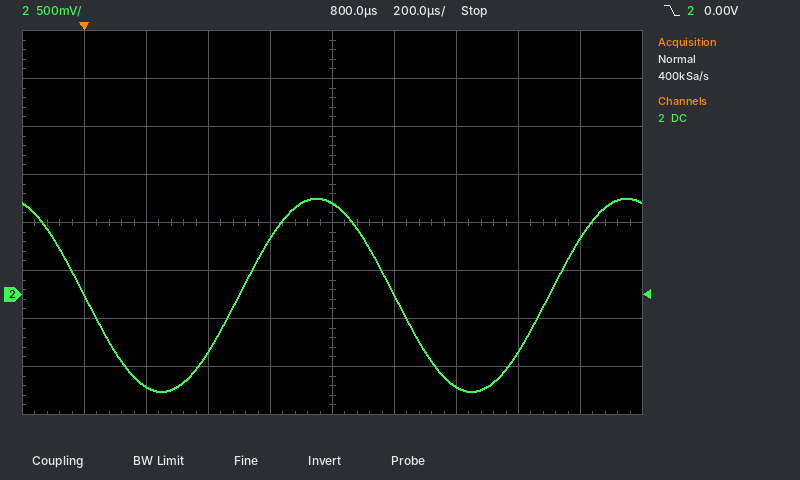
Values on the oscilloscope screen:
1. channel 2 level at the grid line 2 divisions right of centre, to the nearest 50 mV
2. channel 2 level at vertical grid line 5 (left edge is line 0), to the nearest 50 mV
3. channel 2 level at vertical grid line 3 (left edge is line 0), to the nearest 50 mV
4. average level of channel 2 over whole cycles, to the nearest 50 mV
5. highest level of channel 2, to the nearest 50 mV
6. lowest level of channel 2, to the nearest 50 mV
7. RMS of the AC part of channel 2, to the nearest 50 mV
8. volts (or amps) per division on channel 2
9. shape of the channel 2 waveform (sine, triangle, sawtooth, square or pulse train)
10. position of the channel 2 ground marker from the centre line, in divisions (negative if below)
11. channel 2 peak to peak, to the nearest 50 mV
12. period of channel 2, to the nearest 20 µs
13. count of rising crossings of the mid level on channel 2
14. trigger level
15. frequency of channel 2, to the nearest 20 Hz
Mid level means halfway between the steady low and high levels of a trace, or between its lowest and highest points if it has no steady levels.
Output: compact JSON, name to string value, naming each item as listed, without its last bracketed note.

{"channel 2 level at the grid line 2 divisions right of centre, to the nearest 50 mV": "-950 mV", "channel 2 level at vertical grid line 5 (left edge is line 0), to the nearest 50 mV": "950 mV", "channel 2 level at vertical grid line 3 (left edge is line 0), to the nearest 50 mV": "-600 mV", "average level of channel 2 over whole cycles, to the nearest 50 mV": "0 mV", "highest level of channel 2, to the nearest 50 mV": "1.00 V", "lowest level of channel 2, to the nearest 50 mV": "-1.00 V", "RMS of the AC part of channel 2, to the nearest 50 mV": "700 mV", "volts (or amps) per division on channel 2": "500 mV", "shape of the channel 2 waveform": "sine", "position of the channel 2 ground marker from the centre line, in divisions": "-1.5 div", "channel 2 peak to peak, to the nearest 50 mV": "2.00 V", "period of channel 2, to the nearest 20 µs": "1.00 ms", "count of rising crossings of the mid level on channel 2": "2", "trigger level": "0.00 V", "frequency of channel 2, to the nearest 20 Hz": "1.00 kHz"}
